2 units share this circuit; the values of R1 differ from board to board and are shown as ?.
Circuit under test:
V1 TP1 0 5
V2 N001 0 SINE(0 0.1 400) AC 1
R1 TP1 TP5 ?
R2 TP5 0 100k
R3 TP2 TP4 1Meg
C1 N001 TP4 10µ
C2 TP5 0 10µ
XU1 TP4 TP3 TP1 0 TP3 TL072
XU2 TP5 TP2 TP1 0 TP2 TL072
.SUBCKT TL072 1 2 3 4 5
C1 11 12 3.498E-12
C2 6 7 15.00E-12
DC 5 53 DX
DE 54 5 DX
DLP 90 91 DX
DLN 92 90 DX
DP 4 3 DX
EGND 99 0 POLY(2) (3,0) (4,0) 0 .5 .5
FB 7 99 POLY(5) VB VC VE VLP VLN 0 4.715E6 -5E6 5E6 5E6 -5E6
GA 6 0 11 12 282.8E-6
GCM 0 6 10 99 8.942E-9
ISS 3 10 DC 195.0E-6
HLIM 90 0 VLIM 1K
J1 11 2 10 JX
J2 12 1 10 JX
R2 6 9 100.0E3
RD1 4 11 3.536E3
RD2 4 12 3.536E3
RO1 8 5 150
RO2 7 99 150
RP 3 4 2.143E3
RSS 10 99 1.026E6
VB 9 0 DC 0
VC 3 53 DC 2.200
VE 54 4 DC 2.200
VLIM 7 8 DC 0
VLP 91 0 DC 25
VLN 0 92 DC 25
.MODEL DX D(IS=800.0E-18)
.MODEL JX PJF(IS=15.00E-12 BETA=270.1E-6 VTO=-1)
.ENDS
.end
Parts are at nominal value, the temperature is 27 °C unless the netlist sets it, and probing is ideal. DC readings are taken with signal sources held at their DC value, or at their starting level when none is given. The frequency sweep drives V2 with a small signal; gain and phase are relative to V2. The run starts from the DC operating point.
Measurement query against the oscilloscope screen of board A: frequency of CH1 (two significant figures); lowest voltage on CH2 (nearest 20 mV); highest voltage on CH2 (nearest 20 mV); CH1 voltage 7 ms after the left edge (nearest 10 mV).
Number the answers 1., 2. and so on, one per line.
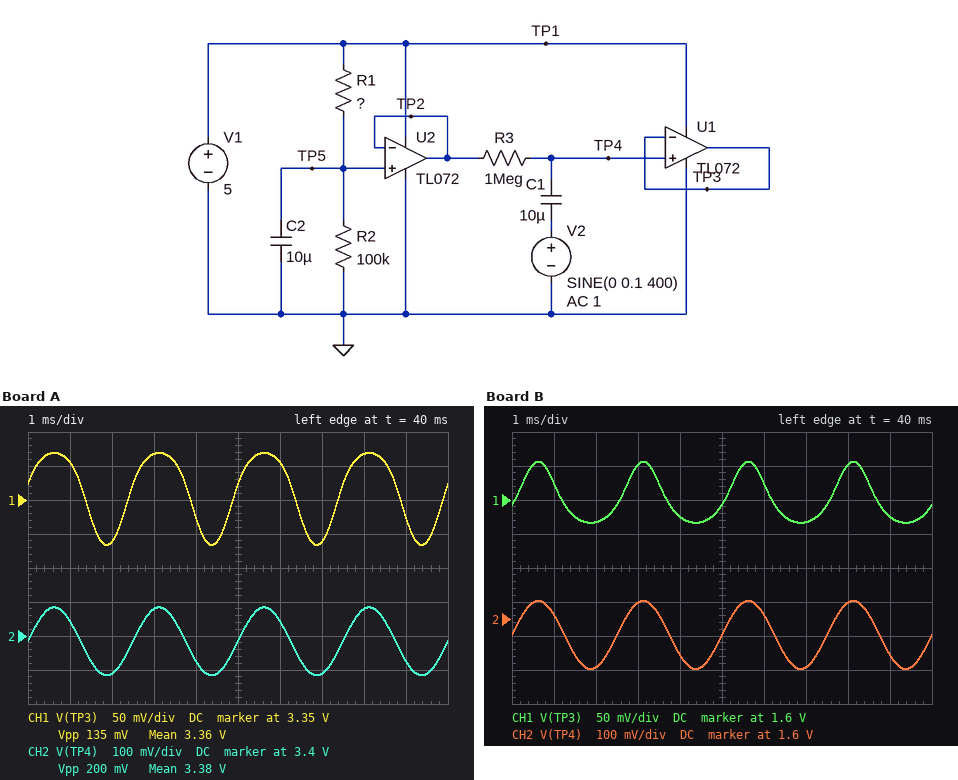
1. 400 Hz
2. 3.28 V
3. 3.48 V
4. 3.29 V
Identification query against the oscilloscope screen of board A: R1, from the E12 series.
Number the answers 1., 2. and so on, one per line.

1. 47 kΩ
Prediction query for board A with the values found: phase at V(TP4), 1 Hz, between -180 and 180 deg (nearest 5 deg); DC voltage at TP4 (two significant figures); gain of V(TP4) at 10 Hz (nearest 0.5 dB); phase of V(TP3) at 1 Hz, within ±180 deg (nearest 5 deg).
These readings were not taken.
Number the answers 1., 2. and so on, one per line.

1. 0 deg
2. 3.4 V
3. 0 dB
4. 0 deg
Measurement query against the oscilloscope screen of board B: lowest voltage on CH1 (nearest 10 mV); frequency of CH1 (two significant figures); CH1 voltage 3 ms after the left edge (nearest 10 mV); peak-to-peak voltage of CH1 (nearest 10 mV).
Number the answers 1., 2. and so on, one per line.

1. 1.57 V
2. 400 Hz
3. 1.65 V
4. 90 mV
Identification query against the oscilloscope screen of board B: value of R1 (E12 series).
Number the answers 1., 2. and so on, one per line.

1. 270 kΩ
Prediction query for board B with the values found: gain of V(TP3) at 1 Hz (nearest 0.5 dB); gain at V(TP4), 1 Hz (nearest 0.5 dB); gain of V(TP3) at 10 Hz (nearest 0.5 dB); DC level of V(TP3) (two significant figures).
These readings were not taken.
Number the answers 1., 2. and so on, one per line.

1. -8.0 dB
2. 0 dB
3. -8.0 dB
4. 1.6 V
